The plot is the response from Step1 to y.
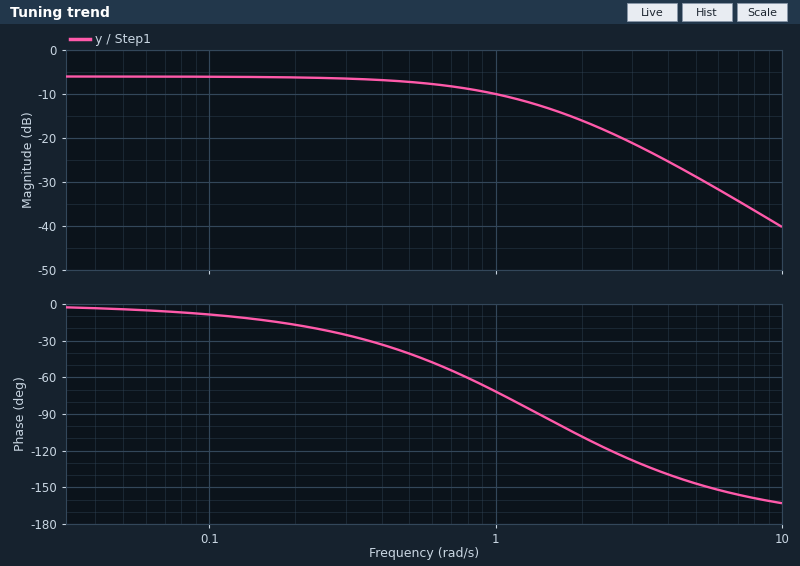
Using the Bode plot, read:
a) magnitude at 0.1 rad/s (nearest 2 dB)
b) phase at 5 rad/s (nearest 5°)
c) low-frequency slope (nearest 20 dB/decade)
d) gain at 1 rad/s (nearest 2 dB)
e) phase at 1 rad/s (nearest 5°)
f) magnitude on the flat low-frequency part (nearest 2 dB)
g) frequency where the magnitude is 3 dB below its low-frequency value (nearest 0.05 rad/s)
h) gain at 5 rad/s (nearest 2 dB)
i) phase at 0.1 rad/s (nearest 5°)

-6 dB
-145°
0 dB/decade
-10 dB
-70°
-6 dB
0.85 rad/s
-28 dB
-10°
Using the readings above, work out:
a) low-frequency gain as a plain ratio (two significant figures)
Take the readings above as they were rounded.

0.50
